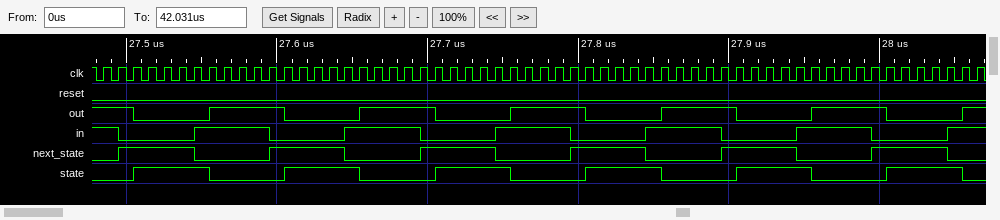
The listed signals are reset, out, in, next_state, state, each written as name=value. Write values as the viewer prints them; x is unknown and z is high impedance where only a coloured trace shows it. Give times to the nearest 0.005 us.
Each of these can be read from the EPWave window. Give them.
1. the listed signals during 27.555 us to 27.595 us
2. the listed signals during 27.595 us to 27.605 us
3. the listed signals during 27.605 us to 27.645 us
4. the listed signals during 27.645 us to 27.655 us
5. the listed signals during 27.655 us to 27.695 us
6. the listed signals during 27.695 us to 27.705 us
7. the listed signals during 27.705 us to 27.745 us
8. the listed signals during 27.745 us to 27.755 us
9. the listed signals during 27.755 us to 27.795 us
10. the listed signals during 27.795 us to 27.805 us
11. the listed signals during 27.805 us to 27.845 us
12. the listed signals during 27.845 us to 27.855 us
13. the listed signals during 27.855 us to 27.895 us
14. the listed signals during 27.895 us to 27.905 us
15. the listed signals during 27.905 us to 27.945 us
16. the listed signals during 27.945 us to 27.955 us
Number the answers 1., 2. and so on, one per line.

1. reset=0, out=1, in=1, next_state=0, state=0
2. reset=0, out=1, in=0, next_state=1, state=0
3. reset=0, out=0, in=0, next_state=1, state=1
4. reset=0, out=0, in=1, next_state=0, state=1
5. reset=0, out=1, in=1, next_state=0, state=0
6. reset=0, out=1, in=0, next_state=1, state=0
7. reset=0, out=0, in=0, next_state=1, state=1
8. reset=0, out=0, in=1, next_state=0, state=1
9. reset=0, out=1, in=1, next_state=0, state=0
10. reset=0, out=1, in=0, next_state=1, state=0
11. reset=0, out=0, in=0, next_state=1, state=1
12. reset=0, out=0, in=1, next_state=0, state=1
13. reset=0, out=1, in=1, next_state=0, state=0
14. reset=0, out=1, in=0, next_state=1, state=0
15. reset=0, out=0, in=0, next_state=1, state=1
16. reset=0, out=0, in=1, next_state=0, state=1
